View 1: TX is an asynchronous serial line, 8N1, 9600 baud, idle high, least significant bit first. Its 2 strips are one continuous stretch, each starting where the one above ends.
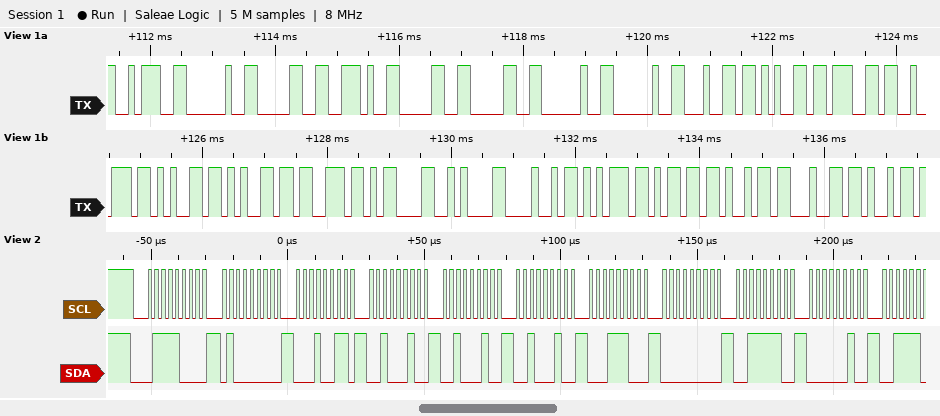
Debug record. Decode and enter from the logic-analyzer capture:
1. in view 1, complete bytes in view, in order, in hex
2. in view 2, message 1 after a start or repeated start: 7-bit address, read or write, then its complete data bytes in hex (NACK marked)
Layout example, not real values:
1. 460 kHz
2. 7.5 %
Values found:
1. 3A 20 30 2E 30 30 20 20 64 65 67 72 65 65 73 0D 0A 48 75 6D 69 64 69
2. 0x3C write: 40 13 22 22 22 1C 00 3E 02
